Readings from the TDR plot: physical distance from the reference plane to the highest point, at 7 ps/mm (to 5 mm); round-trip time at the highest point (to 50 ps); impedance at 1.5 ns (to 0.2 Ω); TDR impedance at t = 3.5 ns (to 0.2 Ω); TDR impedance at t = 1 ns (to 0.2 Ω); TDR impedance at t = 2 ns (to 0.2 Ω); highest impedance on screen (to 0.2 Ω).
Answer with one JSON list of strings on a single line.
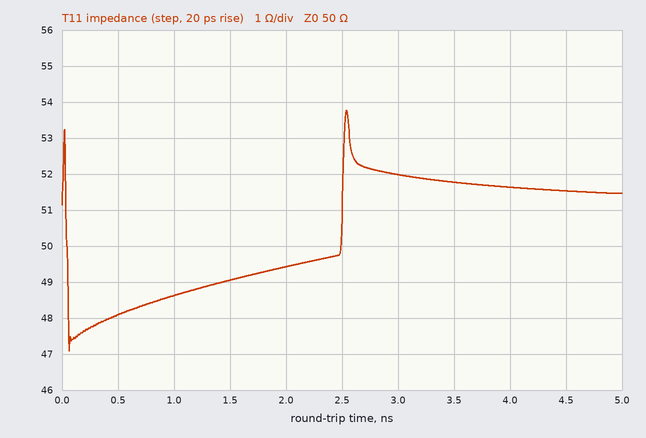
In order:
["180 mm", "2.55 ns", "49.0 Ω", "51.8 Ω", "48.6 Ω", "49.4 Ω", "53.8 Ω"]
